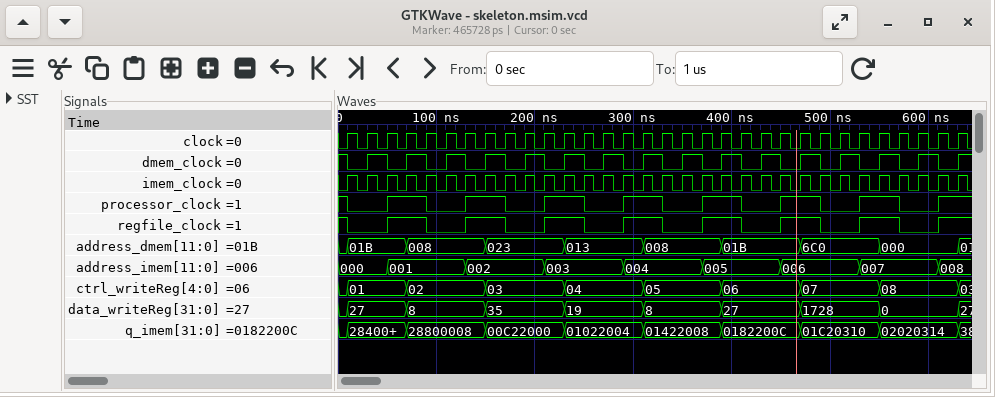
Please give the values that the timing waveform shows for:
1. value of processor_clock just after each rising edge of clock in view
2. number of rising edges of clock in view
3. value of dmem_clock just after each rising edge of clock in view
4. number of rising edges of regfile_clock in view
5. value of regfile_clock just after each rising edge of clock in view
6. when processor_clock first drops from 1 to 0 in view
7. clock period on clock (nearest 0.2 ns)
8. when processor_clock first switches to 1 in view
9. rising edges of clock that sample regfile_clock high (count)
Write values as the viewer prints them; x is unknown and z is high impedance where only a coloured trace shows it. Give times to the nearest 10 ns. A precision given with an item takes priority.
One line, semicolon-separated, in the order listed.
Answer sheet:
0 0 1 1 0 0 1 1 0 0 1 1 0 0 1 1 0 0 1 1 0 0 1 1 0 0 1 1 0 0 1 1; 32; 0 1 0 1 0 1 0 1 0 1 0 1 0 1 0 1 0 1 0 1 0 1 0 1 0 1 0 1 0 1 0 1; 8; 0 0 1 1 0 0 1 1 0 0 1 1 0 0 1 1 0 0 1 1 0 0 1 1 0 0 1 1 0 0 1 1; 10 ns; 20 ns; 50 ns; 16
